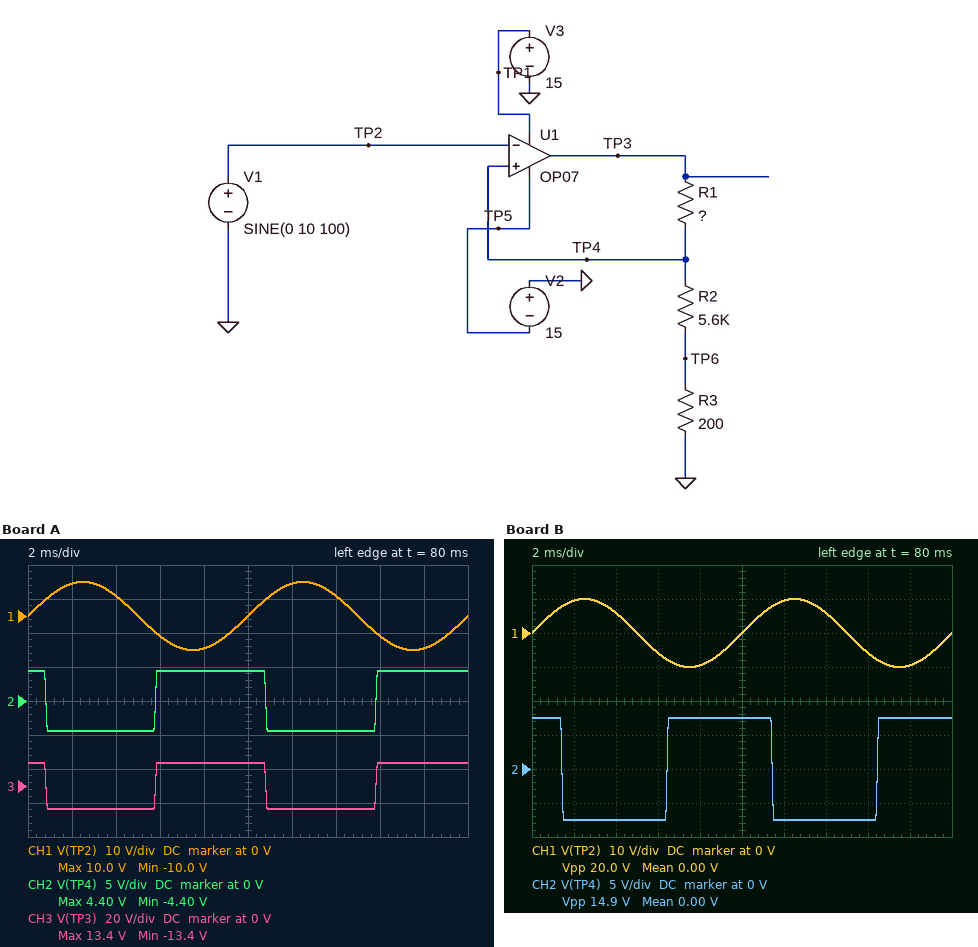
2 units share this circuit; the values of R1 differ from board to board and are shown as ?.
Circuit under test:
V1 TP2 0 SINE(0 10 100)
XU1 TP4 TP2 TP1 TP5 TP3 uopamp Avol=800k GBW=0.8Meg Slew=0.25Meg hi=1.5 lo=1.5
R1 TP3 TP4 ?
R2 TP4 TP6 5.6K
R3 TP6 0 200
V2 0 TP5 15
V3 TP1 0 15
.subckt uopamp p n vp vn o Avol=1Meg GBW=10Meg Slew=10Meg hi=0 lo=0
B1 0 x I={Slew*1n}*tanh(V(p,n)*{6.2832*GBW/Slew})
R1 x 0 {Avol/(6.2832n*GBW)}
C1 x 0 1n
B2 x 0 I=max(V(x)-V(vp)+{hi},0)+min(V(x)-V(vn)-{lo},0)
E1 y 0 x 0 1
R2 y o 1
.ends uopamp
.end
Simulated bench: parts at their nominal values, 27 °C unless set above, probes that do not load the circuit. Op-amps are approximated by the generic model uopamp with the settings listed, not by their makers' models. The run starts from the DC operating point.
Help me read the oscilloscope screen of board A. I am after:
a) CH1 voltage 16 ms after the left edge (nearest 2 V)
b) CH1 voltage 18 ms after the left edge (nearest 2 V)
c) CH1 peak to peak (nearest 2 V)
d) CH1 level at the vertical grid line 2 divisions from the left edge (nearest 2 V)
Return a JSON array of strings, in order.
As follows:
["-6 V", "-10 V", "20 V", "6 V"]
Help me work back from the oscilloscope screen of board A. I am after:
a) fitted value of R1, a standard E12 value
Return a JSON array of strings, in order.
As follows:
["12 kΩ"]
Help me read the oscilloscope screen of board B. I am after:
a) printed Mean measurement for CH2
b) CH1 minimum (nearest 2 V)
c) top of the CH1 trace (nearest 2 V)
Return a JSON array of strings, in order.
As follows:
["0.00 V", "-10 V", "10 V"]
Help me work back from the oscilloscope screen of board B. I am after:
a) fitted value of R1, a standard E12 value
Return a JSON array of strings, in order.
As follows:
["4.7 kΩ"]
